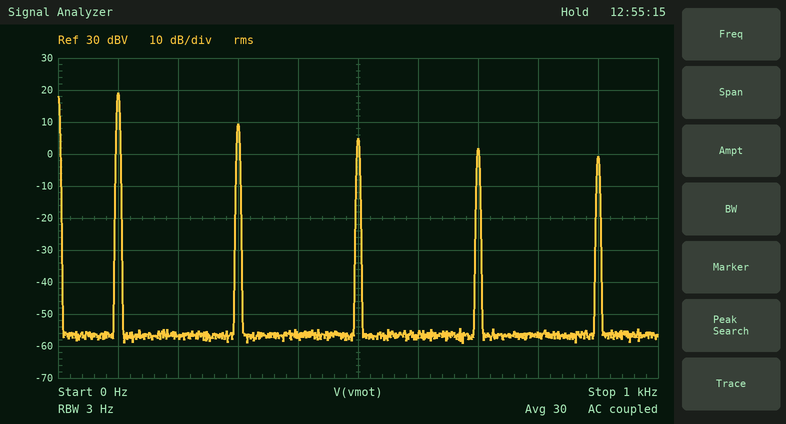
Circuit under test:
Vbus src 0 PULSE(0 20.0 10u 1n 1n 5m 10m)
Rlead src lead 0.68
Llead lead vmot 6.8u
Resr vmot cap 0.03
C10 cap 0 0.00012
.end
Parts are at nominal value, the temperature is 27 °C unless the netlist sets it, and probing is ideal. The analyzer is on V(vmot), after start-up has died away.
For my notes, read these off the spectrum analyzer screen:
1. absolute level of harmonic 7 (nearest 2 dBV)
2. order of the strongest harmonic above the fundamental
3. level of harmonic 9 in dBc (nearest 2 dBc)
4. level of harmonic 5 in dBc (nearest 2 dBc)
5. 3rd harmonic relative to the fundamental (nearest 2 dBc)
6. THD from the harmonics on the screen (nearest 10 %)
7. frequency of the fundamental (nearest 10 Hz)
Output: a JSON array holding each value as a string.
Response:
["2 dBV", "3", "-20 dBc", "-14 dBc", "-10 dBc", "40 %", "100 Hz"]
